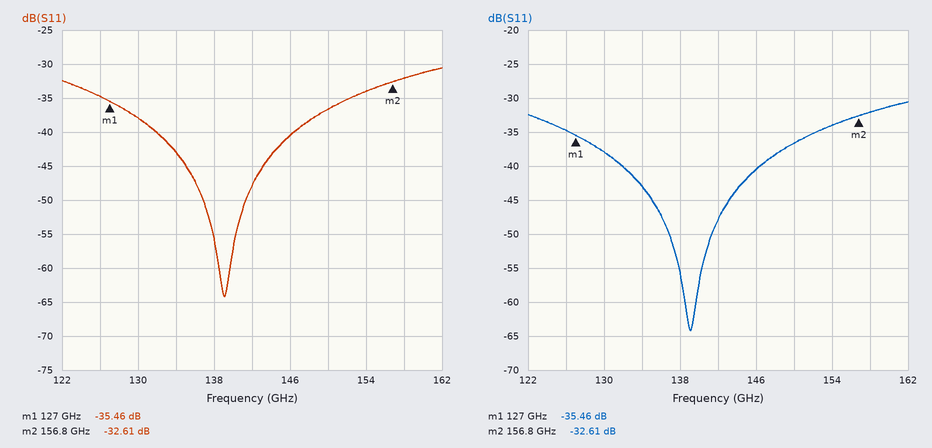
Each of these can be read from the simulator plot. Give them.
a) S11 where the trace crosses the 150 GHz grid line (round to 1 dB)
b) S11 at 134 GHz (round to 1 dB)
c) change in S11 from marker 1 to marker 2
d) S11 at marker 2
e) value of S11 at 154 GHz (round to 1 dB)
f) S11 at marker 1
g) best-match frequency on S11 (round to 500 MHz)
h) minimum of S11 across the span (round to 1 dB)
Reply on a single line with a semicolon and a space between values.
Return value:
-37 dB; -43 dB; 2.85 dB; -32.61 dB; -34 dB; -35.46 dB; 139.0 GHz; -64 dB
